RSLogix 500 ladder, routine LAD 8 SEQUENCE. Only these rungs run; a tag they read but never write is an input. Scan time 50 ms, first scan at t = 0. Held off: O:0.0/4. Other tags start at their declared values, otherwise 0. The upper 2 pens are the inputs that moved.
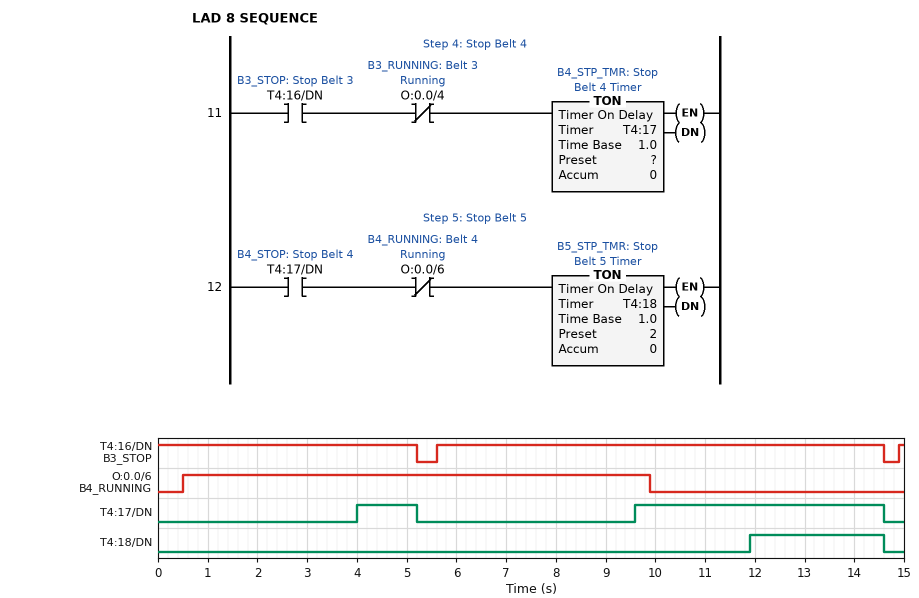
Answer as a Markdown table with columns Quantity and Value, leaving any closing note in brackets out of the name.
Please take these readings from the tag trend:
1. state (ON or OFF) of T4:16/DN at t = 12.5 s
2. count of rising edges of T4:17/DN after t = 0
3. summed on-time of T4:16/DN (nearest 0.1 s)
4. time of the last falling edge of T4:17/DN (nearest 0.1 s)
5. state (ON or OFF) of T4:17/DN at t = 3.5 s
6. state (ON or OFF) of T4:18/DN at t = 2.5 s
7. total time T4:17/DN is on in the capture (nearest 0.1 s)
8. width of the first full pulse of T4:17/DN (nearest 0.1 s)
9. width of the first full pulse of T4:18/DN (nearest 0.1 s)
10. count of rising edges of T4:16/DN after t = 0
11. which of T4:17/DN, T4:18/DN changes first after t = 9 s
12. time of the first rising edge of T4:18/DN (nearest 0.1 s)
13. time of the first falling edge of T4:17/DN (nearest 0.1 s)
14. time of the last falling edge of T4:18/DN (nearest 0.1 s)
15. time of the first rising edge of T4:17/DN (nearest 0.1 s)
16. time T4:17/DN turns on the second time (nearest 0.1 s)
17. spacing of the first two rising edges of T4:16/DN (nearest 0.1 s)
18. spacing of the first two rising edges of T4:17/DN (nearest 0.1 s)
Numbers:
| Quantity | Value |
|---|---|
| state (ON or OFF) of T4:16/DN at t = 12.5 s | ON |
| count of rising edges of T4:17/DN after t = 0 | 2 |
| summed on-time of T4:16/DN | 14.3 s |
| time of the last falling edge of T4:17/DN | 14.6 s |
| state (ON or OFF) of T4:17/DN at t = 3.5 s | OFF |
| state (ON or OFF) of T4:18/DN at t = 2.5 s | OFF |
| total time T4:17/DN is on in the capture | 6.2 s |
| width of the first full pulse of T4:17/DN | 1.2 s |
| width of the first full pulse of T4:18/DN | 2.7 s |
| count of rising edges of T4:16/DN after t = 0 | 2 |
| which of T4:17/DN, T4:18/DN changes first after t = 9 s | T4:17/DN |
| time of the first rising edge of T4:18/DN | 11.9 s |
| time of the first falling edge of T4:17/DN | 5.2 s |
| time of the last falling edge of T4:18/DN | 14.6 s |
| time of the first rising edge of T4:17/DN | 4.0 s |
| time T4:17/DN turns on the second time | 9.6 s |
| spacing of the first two rising edges of T4:16/DN | 9.3 s |
| spacing of the first two rising edges of T4:17/DN | 5.6 s |
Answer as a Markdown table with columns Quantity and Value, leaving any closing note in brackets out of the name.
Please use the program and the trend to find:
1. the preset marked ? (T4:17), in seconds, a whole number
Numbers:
| Quantity | Value |
|---|---|
| the preset marked ? (T4:17), in seconds, a whole number | 4 s |
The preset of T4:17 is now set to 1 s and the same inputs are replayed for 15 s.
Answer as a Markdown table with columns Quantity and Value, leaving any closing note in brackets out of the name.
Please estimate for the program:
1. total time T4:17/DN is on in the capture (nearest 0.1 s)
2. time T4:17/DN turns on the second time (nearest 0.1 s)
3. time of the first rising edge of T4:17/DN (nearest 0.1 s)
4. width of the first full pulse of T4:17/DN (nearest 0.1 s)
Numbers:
| Quantity | Value |
|---|---|
| total time T4:17/DN is on in the capture | 12.2 s |
| time T4:17/DN turns on the second time | 6.6 s |
| time of the first rising edge of T4:17/DN | 1.0 s |
| width of the first full pulse of T4:17/DN | 4.2 s |
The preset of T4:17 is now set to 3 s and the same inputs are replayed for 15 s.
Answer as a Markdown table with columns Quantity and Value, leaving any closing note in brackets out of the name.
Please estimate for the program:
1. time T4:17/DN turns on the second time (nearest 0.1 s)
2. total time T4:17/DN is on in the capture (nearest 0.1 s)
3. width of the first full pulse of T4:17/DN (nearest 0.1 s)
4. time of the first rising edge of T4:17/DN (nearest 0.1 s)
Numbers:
| Quantity | Value |
|---|---|
| time T4:17/DN turns on the second time | 8.6 s |
| total time T4:17/DN is on in the capture | 8.2 s |
| width of the first full pulse of T4:17/DN | 2.2 s |
| time of the first rising edge of T4:17/DN | 3.0 s |
